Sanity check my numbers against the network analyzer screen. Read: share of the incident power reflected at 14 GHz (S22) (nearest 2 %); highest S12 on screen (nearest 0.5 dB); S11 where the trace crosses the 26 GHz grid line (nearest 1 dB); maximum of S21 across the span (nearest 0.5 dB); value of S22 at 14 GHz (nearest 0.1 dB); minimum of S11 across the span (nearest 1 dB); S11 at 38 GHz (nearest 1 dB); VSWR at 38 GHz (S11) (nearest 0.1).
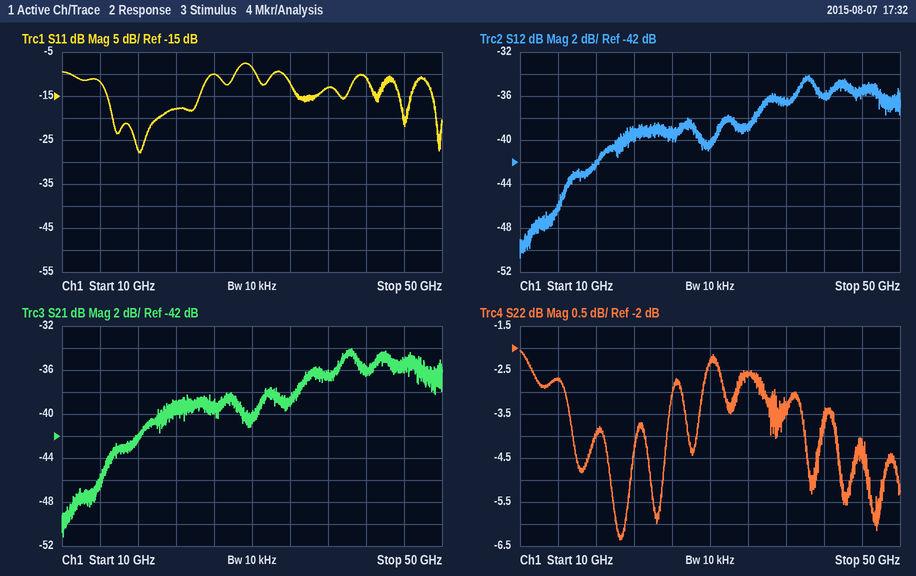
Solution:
54 %
-34.0 dB
-10 dB
-34.0 dB
-2.7 dB
-28 dB
-13 dB
1.6
